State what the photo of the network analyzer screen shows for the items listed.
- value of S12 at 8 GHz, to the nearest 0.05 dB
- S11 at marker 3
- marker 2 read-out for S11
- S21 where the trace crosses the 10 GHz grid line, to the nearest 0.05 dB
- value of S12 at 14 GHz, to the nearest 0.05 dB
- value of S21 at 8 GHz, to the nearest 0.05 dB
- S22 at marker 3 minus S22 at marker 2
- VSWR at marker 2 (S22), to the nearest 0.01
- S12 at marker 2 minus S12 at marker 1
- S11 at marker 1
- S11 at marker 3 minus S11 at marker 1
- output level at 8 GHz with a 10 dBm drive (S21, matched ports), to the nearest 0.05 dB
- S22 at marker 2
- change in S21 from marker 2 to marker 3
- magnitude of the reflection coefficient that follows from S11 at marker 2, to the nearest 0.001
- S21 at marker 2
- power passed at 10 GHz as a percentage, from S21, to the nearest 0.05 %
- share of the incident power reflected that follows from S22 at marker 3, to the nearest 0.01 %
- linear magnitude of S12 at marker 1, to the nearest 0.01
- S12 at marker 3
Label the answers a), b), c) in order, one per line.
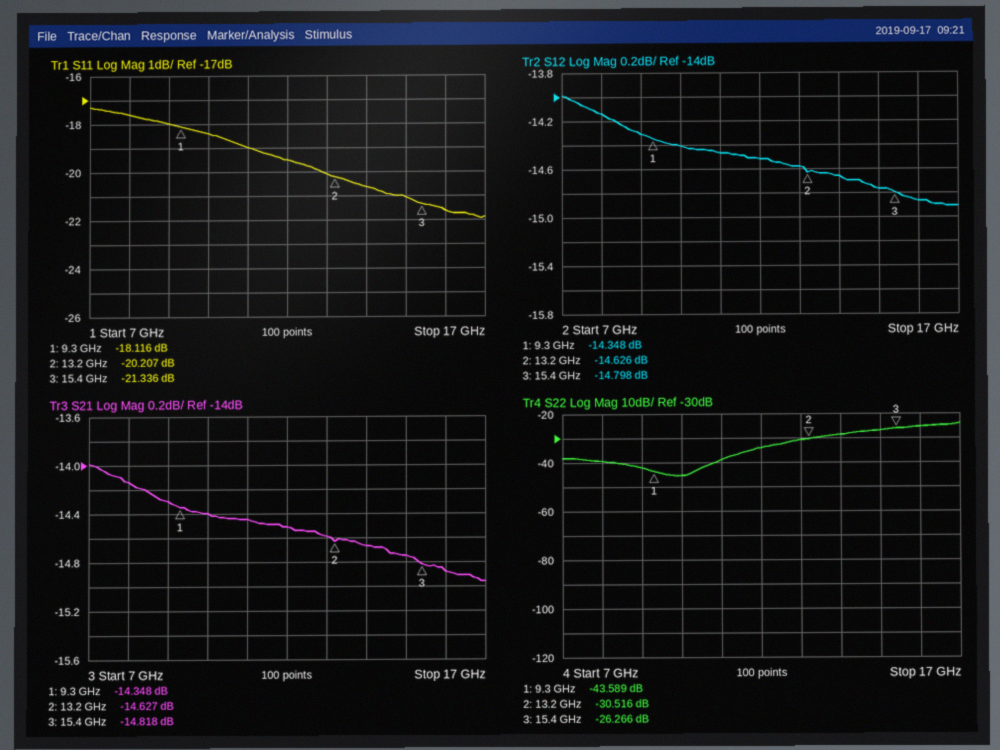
a) -14.15 dB
b) -21.336 dB
c) -20.207 dB
d) -14.40 dB
e) -14.65 dB
f) -14.15 dB
g) 4.250 dB
h) 1.06
i) -0.278 dB
j) -18.116 dB
k) -3.220 dB
l) -4.15 dBm
m) -30.516 dB
n) -0.191 dB
o) 0.098
p) -14.627 dB
q) 3.65 %
r) 0.24 %
s) 0.19
t) -14.798 dB
